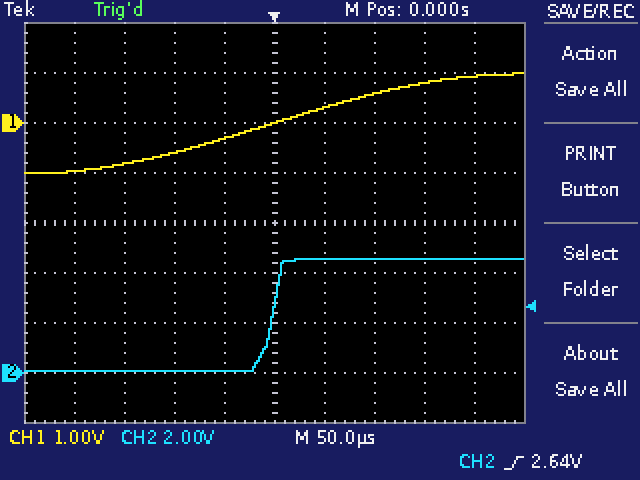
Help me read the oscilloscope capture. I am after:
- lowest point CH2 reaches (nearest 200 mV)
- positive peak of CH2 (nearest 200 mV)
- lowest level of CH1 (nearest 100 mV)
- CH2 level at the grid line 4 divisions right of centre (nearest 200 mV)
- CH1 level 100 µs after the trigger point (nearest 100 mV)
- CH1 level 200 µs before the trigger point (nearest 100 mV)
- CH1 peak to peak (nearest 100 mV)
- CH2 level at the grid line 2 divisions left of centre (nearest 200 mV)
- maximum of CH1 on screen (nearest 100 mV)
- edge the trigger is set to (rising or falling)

0.0 V
4.6 V
-1.0 V
4.6 V
600 mV
-1.0 V
2.0 V
0.0 V
1.0 V
rising
